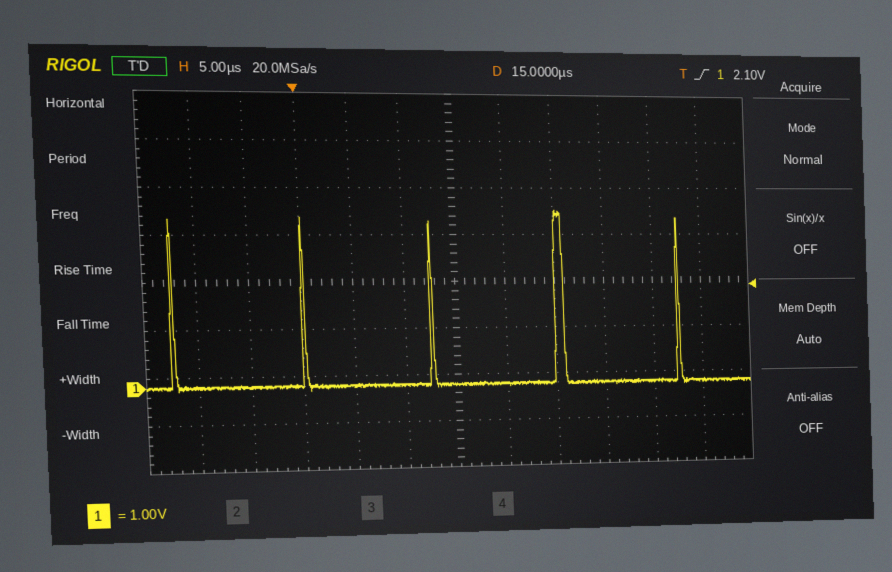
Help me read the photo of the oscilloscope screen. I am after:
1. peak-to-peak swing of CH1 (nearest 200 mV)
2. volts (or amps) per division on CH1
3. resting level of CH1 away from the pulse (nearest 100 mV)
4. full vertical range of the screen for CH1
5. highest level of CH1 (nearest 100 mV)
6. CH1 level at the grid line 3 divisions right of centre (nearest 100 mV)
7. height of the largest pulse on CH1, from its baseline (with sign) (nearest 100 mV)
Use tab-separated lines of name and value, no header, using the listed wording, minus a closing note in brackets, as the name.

peak-to-peak swing of CH1	3.8 V
volts (or amps) per division on CH1	1 V
resting level of CH1 away from the pulse	0.0 V
full vertical range of the screen for CH1	8 V
highest level of CH1	3.7 V
CH1 level at the grid line 3 divisions right of centre	0.0 V
height of the largest pulse on CH1, from its baseline (with sign)	+3.7 V
